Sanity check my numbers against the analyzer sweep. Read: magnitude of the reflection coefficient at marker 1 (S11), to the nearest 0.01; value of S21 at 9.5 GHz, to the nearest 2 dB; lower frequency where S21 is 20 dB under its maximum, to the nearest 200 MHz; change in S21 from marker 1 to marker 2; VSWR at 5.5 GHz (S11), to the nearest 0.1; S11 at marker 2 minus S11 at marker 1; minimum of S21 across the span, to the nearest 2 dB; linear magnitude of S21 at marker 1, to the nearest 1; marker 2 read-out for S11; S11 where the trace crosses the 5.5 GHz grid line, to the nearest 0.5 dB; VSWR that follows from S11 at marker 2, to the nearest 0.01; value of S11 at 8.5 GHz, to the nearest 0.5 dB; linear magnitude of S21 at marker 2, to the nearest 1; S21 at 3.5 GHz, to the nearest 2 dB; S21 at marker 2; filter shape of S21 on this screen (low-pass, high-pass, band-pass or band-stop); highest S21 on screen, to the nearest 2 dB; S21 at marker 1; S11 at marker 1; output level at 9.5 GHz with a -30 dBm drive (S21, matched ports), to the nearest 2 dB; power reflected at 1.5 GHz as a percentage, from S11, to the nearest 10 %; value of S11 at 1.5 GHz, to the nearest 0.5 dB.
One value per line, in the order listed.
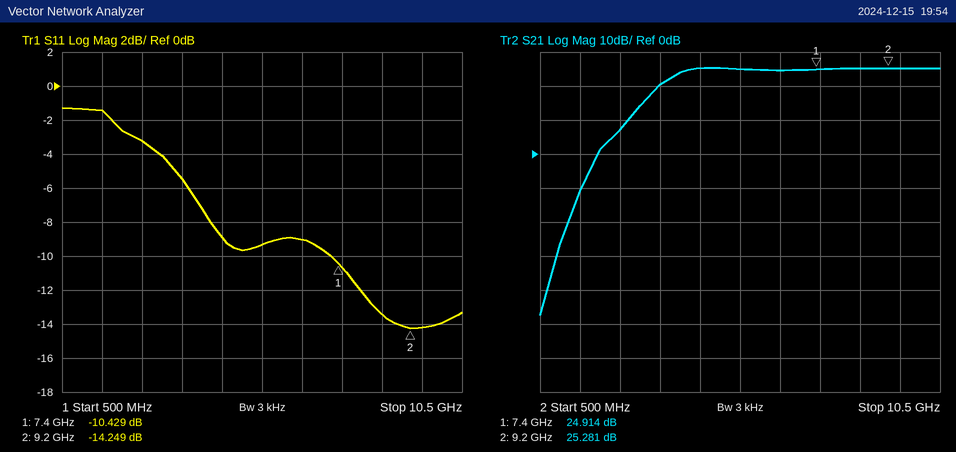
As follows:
0.30
26 dB
2.4 GHz
0.367 dB
2.0
-3.820 dB
-48 dB
18
-14.249 dB
-9.5 dB
1.48
-13.5 dB
18
20 dB
25.281 dB
high-pass
26 dB
24.914 dB
-10.429 dB
-4 dBm
70 %
-1.5 dB
